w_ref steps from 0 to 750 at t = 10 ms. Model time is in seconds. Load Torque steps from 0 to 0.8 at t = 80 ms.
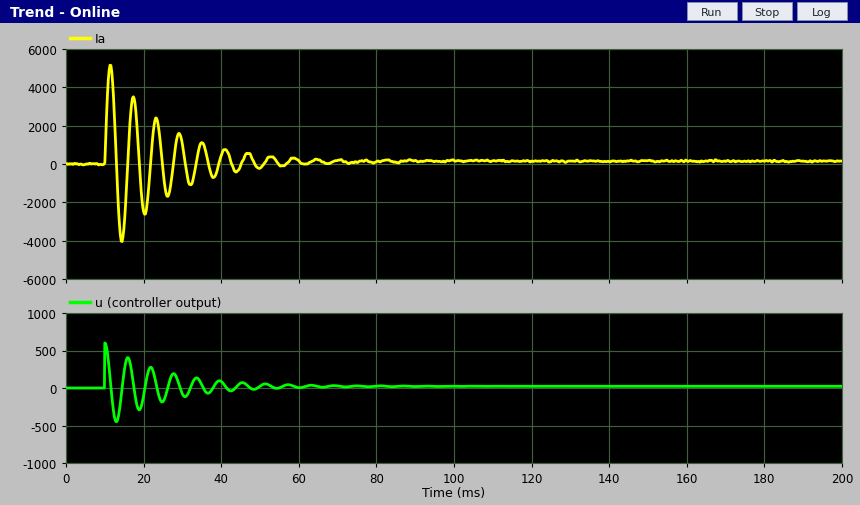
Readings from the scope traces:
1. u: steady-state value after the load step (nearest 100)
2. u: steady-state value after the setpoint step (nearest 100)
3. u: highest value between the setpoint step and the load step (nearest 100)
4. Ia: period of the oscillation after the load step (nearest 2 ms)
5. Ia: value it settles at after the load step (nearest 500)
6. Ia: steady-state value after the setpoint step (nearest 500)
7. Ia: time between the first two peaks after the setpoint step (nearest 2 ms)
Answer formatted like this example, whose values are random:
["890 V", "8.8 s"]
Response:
["0", "0", "600", "6 ms", "0", "0", "6 ms"]
